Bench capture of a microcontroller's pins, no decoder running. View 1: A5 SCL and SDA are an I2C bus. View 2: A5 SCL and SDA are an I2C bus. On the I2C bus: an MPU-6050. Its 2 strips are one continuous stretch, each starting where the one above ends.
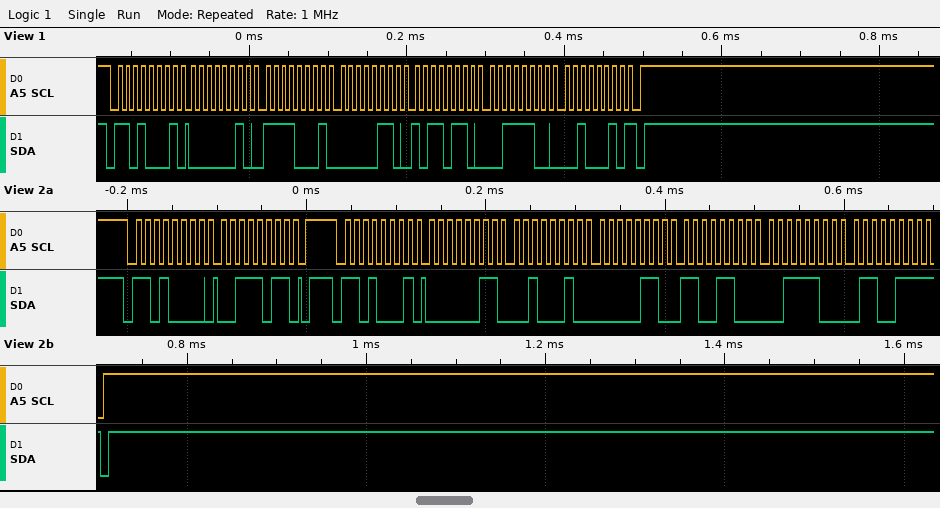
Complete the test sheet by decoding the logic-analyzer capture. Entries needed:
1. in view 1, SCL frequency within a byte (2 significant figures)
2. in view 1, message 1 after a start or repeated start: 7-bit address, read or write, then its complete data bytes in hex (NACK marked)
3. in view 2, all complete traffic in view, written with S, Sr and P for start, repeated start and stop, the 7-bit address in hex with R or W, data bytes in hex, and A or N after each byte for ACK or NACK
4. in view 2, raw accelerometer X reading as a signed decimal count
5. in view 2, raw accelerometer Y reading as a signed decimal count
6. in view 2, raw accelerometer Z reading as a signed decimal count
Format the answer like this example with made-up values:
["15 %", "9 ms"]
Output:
["100 kHz", "0x68 read: 02 F1 06 B6 3C 22 NACK", "S 68W A 3B A P S 68R A 03 A 22 A 06 A CC A 3C A 67 N P", "802", "1740", "15463"]
